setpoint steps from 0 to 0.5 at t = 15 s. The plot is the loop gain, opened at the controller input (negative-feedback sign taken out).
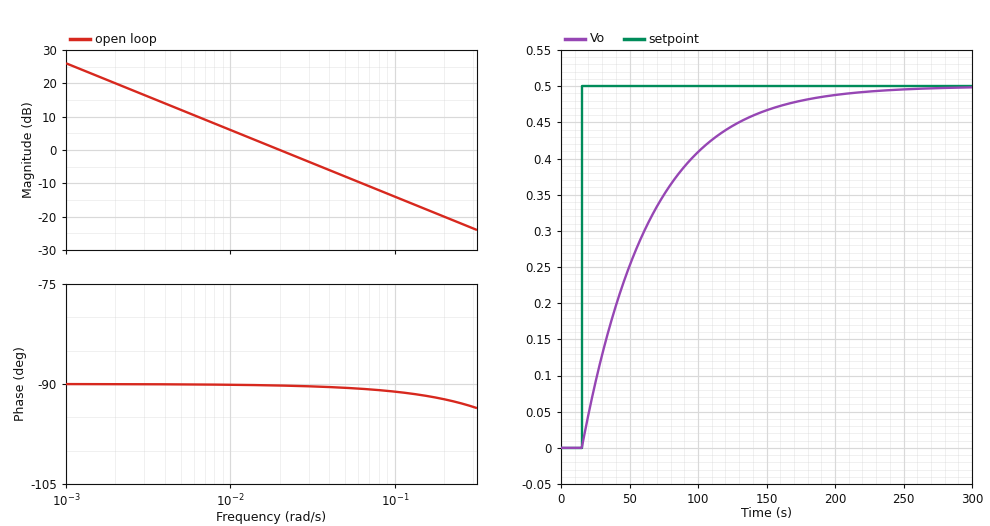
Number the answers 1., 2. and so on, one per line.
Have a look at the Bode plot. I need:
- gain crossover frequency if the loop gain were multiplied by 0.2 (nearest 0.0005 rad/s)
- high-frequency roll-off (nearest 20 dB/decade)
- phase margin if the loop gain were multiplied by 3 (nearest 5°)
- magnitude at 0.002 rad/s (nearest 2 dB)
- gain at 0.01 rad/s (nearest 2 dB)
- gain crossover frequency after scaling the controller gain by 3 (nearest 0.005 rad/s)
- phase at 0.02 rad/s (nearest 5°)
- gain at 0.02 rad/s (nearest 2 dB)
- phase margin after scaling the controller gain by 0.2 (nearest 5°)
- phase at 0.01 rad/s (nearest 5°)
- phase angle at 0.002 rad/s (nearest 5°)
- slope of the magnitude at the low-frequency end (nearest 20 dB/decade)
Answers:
1. 0.0040 rad/s
2. -20 dB/decade
3. 90°
4. 20 dB
5. 6 dB
6. 0.060 rad/s
7. -90°
8. 0 dB
9. 90°
10. -90°
11. -90°
12. -20 dB/decade
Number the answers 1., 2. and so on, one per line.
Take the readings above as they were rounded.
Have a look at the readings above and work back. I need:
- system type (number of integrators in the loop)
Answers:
1. 1
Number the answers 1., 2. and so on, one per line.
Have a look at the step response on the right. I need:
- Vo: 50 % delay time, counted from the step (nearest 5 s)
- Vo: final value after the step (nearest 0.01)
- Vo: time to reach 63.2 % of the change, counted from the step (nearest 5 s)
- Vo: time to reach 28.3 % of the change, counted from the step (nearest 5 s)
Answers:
1. 35 s
2. 0.50
3. 50 s
4. 15 s
